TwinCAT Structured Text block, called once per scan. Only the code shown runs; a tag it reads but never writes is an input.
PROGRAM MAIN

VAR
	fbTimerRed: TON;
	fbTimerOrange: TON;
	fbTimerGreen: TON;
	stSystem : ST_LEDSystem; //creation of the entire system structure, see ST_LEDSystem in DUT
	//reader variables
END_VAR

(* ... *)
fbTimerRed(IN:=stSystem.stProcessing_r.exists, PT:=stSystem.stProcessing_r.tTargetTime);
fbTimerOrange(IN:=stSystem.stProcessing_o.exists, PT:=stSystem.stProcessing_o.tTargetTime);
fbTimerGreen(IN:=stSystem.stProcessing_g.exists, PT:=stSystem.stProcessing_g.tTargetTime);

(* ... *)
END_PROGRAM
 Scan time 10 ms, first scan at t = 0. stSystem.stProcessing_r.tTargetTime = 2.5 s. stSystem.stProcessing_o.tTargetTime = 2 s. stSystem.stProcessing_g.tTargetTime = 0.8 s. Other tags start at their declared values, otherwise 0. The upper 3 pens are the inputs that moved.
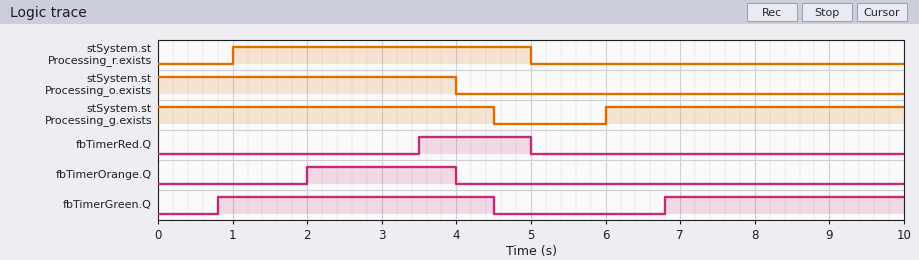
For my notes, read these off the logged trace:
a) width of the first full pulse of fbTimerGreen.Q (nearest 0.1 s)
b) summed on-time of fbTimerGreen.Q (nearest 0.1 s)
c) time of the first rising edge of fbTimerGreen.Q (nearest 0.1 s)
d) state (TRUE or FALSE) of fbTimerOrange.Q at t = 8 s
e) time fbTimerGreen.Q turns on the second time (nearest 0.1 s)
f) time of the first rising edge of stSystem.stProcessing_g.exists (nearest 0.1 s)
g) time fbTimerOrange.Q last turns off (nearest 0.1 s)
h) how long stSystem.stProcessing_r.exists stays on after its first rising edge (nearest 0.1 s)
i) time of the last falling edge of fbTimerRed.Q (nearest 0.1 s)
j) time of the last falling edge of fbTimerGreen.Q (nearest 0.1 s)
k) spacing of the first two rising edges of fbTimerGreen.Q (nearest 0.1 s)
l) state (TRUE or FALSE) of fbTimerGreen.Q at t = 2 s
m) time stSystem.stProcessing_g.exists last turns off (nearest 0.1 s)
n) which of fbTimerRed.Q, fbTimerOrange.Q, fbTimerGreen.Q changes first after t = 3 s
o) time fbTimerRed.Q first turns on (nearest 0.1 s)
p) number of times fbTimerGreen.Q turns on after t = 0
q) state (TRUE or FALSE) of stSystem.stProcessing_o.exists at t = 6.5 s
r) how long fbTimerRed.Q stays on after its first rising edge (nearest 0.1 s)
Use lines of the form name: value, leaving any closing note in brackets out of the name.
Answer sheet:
width of the first full pulse of fbTimerGreen.Q: 3.7 s
summed on-time of fbTimerGreen.Q: 6.9 s
time of the first rising edge of fbTimerGreen.Q: 0.8 s
state (TRUE or FALSE) of fbTimerOrange.Q at t = 8 s: FALSE
time fbTimerGreen.Q turns on the second time: 6.8 s
time of the first rising edge of stSystem.stProcessing_g.exists: 6.0 s
time fbTimerOrange.Q last turns off: 4.0 s
how long stSystem.stProcessing_r.exists stays on after its first rising edge: 4.0 s
time of the last falling edge of fbTimerRed.Q: 5.0 s
time of the last falling edge of fbTimerGreen.Q: 4.5 s
spacing of the first two rising edges of fbTimerGreen.Q: 6.0 s
state (TRUE or FALSE) of fbTimerGreen.Q at t = 2 s: TRUE
time stSystem.stProcessing_g.exists last turns off: 4.5 s
which of fbTimerRed.Q, fbTimerOrange.Q, fbTimerGreen.Q changes first after t = 3 s: fbTimerRed.Q
time fbTimerRed.Q first turns on: 3.5 s
number of times fbTimerGreen.Q turns on after t = 0: 2
state (TRUE or FALSE) of stSystem.stProcessing_o.exists at t = 6.5 s: FALSE
how long fbTimerRed.Q stays on after its first rising edge: 1.5 s
